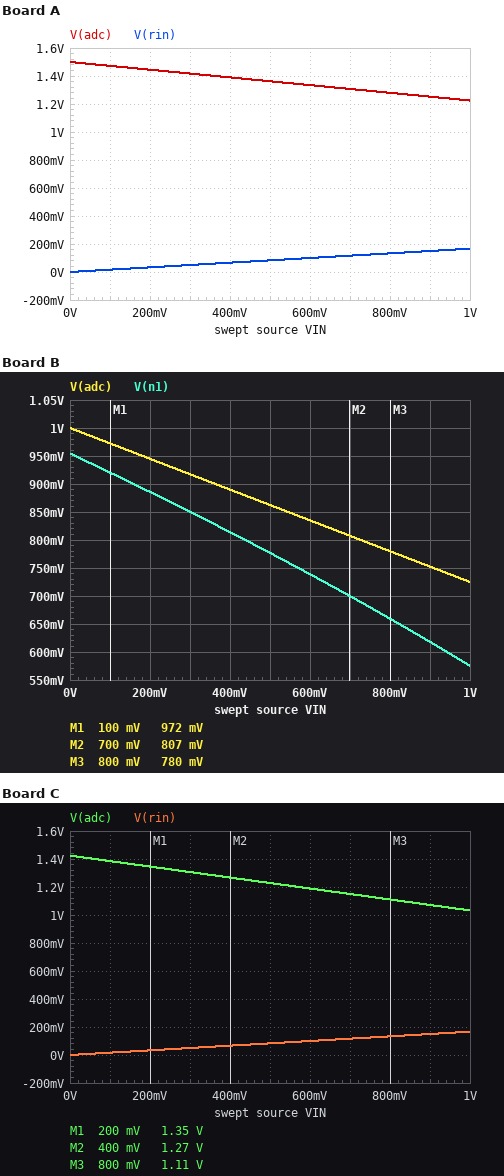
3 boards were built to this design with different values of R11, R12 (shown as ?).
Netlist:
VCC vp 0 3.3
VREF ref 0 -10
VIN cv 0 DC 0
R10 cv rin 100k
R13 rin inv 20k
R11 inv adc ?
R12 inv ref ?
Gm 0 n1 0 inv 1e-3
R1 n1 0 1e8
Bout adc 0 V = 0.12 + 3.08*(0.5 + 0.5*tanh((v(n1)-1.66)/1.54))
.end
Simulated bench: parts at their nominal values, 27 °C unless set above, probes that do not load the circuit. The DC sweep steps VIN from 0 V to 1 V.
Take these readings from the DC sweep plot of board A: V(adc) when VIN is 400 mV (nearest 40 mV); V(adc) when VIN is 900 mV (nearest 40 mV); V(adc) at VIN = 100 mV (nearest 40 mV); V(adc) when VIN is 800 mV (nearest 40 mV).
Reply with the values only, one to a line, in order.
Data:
1.40 V
1.24 V
1.48 V
1.28 V
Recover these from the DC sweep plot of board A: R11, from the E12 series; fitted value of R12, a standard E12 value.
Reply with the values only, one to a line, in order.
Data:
33 kΩ
220 kΩ
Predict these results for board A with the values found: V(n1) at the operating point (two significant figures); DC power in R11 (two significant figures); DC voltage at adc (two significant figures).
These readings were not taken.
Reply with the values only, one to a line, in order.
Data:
1.5 V
68 µW
1.5 V
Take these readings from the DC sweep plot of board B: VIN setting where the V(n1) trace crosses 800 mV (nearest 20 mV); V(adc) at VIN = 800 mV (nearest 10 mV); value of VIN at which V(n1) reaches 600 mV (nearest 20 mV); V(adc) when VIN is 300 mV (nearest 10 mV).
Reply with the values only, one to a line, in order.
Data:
440 mV
780 mV
940 mV
920 mV
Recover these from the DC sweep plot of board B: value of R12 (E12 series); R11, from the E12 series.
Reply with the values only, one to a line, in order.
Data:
330 kΩ
33 kΩ
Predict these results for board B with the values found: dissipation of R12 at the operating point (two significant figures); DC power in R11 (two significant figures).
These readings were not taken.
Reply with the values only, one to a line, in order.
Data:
300 µW
30 µW
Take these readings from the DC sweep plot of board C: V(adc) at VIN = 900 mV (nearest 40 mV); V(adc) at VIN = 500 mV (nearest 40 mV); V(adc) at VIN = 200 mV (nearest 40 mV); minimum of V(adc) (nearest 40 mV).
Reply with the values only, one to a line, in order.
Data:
1.08 V
1.24 V
1.36 V
1.04 V
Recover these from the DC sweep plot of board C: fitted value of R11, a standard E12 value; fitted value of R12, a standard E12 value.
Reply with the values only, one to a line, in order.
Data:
47 kΩ
330 kΩ
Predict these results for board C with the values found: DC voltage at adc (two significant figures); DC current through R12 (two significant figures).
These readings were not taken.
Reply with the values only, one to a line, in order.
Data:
1.4 V
30 µA
